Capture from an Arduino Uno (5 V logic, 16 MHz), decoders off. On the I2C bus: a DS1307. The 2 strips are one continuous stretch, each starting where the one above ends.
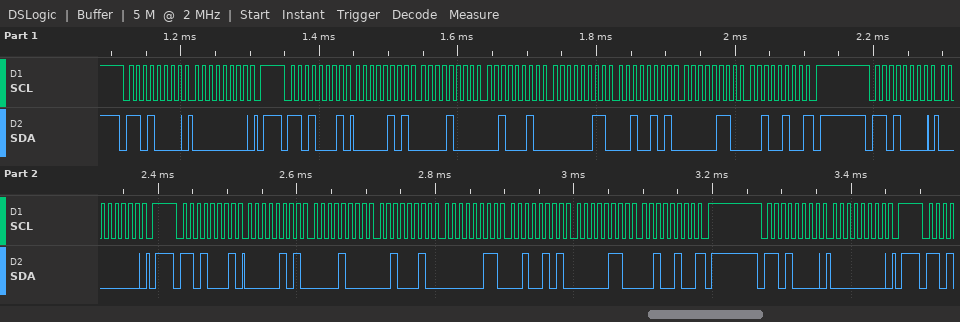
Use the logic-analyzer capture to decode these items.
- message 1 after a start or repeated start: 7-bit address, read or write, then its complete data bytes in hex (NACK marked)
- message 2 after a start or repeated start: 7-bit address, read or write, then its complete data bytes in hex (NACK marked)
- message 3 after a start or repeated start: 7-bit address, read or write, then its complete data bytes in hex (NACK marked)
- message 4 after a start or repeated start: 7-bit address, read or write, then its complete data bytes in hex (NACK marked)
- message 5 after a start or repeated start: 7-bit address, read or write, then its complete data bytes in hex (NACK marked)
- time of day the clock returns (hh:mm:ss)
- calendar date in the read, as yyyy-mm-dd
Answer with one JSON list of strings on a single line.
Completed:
["0x68 write: 00", "0x68 read: 05 08 22 03 25 06 24 NACK", "0x68 write: 00", "0x68 read: 05 08 22 03 25 06 24 NACK", "0x68 write: 00", "22:08:05", "2024-06-25"]
